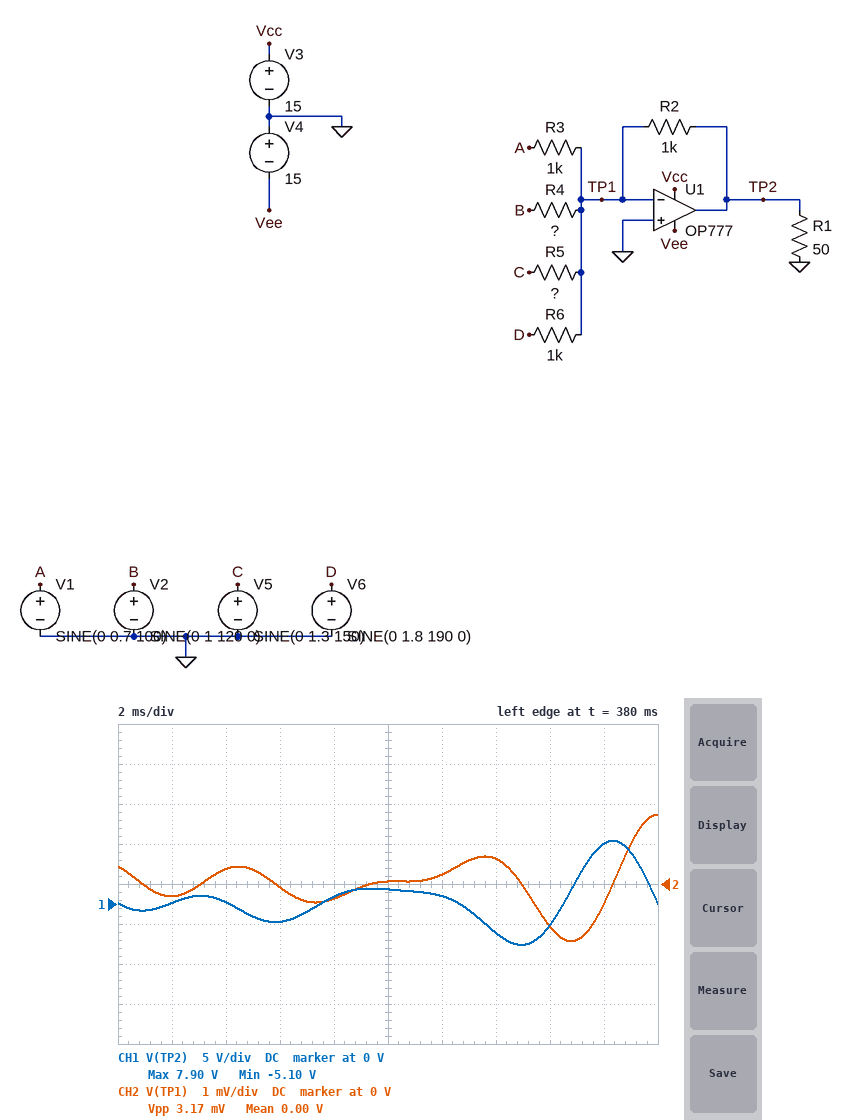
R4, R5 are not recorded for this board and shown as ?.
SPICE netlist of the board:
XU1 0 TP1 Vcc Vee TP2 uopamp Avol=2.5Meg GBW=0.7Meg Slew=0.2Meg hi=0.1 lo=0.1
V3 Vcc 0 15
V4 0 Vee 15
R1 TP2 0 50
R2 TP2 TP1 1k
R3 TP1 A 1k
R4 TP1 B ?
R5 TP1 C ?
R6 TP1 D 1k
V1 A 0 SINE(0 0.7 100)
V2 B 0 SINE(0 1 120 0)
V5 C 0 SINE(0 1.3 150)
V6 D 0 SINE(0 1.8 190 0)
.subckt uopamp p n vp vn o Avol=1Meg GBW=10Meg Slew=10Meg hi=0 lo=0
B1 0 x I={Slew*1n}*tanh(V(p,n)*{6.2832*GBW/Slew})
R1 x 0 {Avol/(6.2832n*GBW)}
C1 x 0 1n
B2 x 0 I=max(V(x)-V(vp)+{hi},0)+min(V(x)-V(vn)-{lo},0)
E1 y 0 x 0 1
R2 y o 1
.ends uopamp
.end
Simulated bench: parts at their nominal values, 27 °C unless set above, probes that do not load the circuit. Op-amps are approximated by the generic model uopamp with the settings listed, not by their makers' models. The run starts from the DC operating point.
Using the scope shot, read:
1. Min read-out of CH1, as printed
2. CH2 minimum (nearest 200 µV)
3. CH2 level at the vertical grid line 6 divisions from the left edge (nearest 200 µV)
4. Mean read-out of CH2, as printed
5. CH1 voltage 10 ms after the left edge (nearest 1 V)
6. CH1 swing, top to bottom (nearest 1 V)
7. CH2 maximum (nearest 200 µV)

-5.10 V
-1.4 mV
200 µV
0.00 V
2 V
13 V
1.8 mV
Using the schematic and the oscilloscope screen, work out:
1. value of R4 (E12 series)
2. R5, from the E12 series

330 Ω
470 Ω
